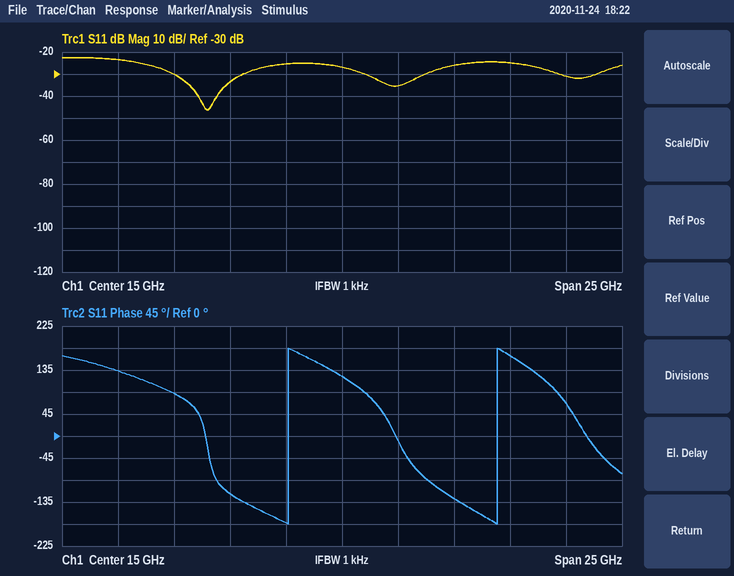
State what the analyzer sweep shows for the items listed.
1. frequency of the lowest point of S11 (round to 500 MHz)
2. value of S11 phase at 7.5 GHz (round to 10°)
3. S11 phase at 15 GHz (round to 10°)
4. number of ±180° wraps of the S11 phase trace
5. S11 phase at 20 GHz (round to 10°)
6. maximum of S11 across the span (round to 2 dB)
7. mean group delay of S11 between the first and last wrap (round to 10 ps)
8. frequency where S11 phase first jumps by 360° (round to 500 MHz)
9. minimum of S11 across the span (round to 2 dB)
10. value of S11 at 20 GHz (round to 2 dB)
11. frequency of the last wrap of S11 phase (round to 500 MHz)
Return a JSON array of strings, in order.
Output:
["9.0 GHz", "90°", "120°", "2", "-130°", "-22 dB", "110 ps", "12.5 GHz", "-46 dB", "-26 dB", "22.0 GHz"]
